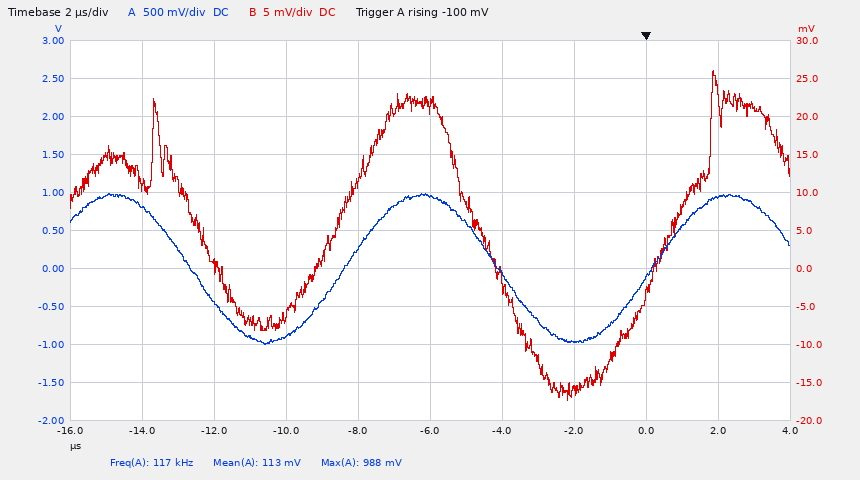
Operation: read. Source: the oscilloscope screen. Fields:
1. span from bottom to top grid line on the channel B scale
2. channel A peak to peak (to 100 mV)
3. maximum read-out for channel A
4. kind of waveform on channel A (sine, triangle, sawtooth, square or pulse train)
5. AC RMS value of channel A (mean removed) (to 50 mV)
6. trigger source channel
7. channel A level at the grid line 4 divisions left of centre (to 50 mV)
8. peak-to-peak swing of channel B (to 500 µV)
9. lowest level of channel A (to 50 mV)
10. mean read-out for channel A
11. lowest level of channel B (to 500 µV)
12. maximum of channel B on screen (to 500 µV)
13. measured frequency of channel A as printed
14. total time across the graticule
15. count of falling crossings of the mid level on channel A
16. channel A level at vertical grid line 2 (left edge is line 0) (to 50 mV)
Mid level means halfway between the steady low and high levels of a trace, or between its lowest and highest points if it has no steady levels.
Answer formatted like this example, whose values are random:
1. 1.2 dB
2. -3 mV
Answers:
1. 50 mV
2. 2.00 V
3. 988 mV
4. sine
5. 700 mV
6. channel A
7. 800 mV
8. 43.5 mV
9. -1.00 V
10. 113 mV
11. -17.5 mV
12. 26.0 mV
13. 117 kHz
14. 20 µs
15. 2
16. -450 mV
